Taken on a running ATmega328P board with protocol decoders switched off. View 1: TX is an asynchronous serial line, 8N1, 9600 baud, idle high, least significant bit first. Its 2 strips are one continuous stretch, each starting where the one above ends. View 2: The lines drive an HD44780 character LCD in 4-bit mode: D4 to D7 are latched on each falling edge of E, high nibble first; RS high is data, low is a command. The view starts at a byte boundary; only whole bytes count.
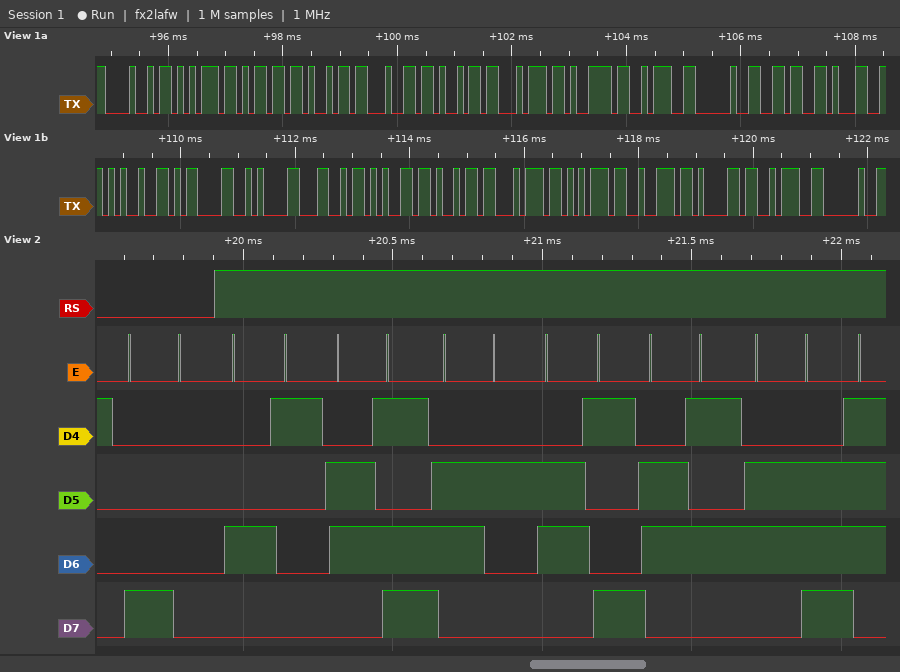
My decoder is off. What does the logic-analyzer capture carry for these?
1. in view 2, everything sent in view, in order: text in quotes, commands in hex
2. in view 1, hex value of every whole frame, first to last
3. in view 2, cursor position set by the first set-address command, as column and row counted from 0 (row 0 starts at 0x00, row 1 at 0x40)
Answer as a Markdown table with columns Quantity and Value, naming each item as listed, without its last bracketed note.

| Quantity | Value |
|---|---|
| in view 2, everything sent in view, in order: text in quotes, commands in hex | 0x80 "Ambien" |
| in view 1, hex value of every whole frame, first to last | 48 75 6D 69 64 69 74 79 3A 20 36 31 25 0D 0A 4C 65 69 74 75 72 61 3A 20 |
| in view 2, cursor position set by the first set-address command, as column and row counted from 0 | column 0, row 0 |
